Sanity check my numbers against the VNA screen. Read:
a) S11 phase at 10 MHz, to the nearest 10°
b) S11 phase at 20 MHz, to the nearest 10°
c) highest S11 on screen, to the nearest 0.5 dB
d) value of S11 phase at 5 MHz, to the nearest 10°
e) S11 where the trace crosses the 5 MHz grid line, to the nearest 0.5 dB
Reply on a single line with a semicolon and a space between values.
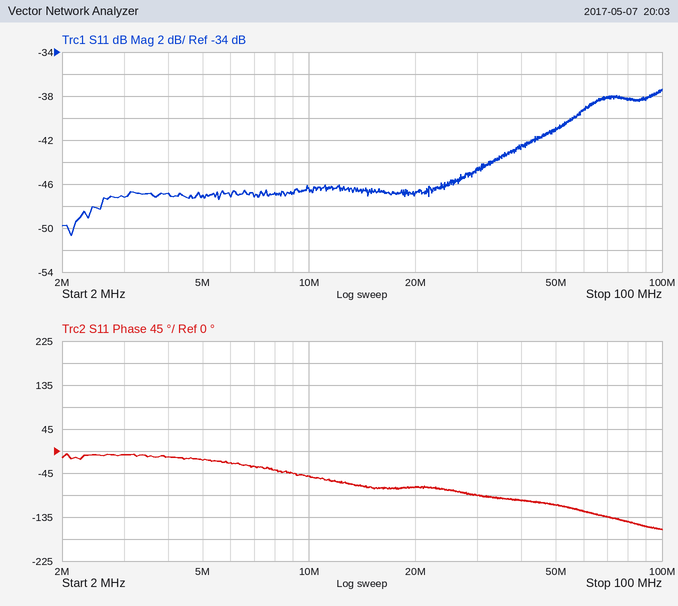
-50°; -70°; -37.5 dB; -20°; -47.0 dB
